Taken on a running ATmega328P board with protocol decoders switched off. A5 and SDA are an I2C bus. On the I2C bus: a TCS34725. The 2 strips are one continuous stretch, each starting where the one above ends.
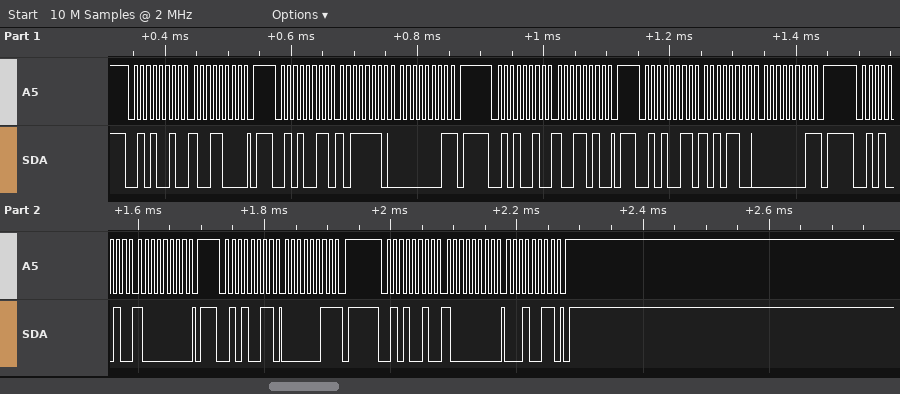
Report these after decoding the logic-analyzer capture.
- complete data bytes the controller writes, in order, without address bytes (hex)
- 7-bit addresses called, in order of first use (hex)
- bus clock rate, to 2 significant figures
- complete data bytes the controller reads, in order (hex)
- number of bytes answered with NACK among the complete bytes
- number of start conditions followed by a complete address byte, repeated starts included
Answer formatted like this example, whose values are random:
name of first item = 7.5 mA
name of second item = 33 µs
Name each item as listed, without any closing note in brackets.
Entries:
complete data bytes the controller writes, in order, without address bytes = 98 9A 80 80 13
7-bit addresses called, in order of first use = 0x29
bus clock rate, to 2 significant figures = 100 kHz
complete data bytes the controller reads, in order = BE 01 AC 01 03
number of bytes answered with NACK among the complete bytes = 3
number of start conditions followed by a complete address byte, repeated starts included = 7
